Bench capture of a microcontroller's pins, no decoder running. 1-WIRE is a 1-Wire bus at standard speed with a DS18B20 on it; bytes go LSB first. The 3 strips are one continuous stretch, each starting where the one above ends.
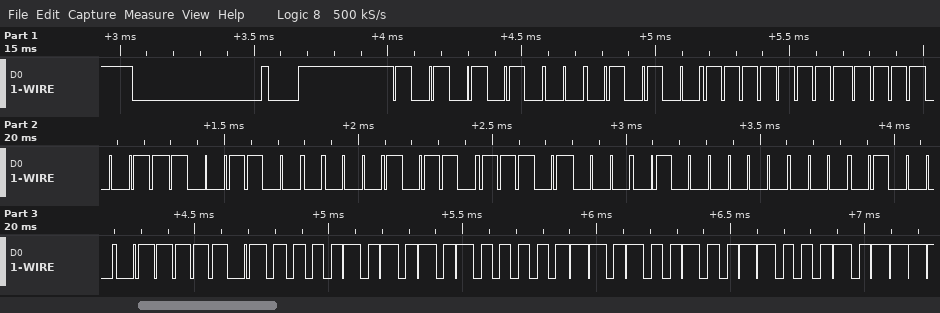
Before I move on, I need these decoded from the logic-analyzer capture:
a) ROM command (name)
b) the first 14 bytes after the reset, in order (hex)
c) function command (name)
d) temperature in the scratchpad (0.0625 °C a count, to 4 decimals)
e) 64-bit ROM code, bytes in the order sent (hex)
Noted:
Match ROM
55 28 FF CF 19 68 17 02 10 BE 50 05 4B 46
Read Scratchpad
85.0000 °C
28 FF CF 19 68 17 02 10
